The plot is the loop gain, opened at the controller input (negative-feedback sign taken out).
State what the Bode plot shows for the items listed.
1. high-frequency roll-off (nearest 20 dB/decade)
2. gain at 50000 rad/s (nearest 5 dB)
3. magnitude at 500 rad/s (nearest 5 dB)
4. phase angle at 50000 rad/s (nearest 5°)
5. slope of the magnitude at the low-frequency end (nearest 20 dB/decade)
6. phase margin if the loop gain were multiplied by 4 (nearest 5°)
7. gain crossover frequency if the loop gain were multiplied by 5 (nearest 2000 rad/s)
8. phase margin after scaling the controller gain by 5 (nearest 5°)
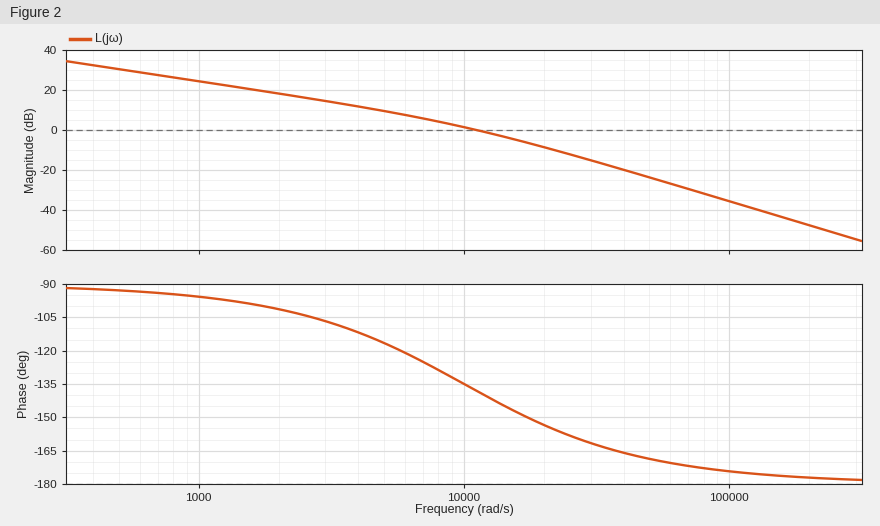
-40 dB/decade
-25 dB
30 dB
-170°
-20 dB/decade
20°
28000 rad/s
20°
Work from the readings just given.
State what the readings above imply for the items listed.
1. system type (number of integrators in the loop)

1
